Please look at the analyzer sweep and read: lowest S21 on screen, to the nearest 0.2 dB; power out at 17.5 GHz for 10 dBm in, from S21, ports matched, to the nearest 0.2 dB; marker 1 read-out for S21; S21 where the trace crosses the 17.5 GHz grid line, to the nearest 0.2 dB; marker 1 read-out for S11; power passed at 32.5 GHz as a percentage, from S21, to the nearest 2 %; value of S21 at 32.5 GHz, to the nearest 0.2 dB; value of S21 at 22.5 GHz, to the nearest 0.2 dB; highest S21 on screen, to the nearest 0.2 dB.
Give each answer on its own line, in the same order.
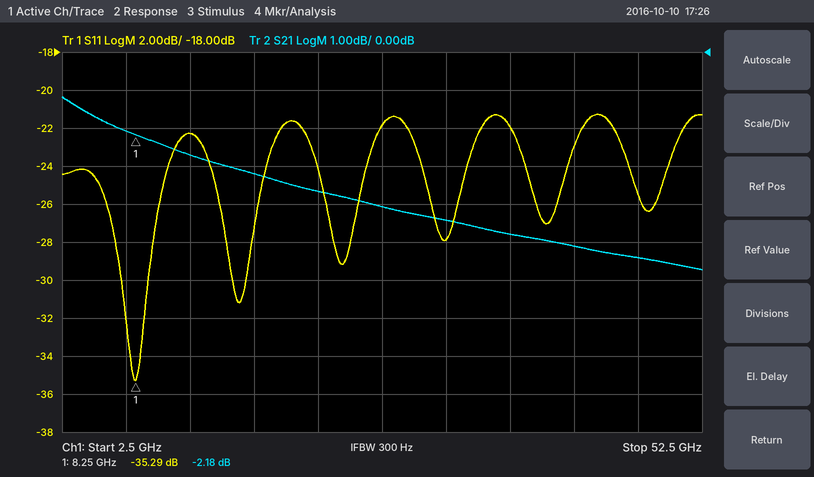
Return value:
-5.8 dB
6.8 dBm
-2.18 dB
-3.2 dB
-35.29 dB
36 %
-4.4 dB
-3.6 dB
-1.2 dB
